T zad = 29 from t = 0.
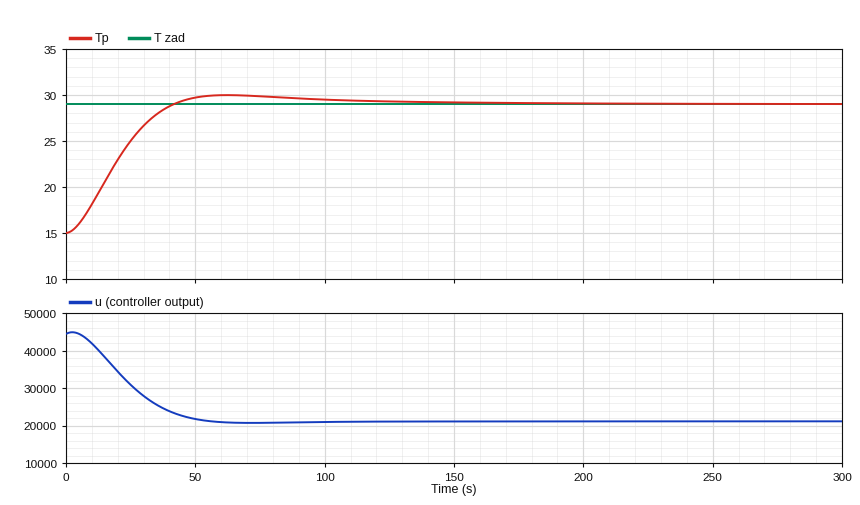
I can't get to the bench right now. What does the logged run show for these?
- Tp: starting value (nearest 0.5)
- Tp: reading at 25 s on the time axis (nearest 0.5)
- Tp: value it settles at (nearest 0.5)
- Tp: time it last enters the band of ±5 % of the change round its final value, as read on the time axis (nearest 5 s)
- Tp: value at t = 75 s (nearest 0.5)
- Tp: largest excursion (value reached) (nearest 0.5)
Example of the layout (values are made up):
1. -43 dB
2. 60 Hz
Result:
1. 15.0
2. 25.0
3. 29.0
4. 85 s
5. 30.0
6. 30.0
